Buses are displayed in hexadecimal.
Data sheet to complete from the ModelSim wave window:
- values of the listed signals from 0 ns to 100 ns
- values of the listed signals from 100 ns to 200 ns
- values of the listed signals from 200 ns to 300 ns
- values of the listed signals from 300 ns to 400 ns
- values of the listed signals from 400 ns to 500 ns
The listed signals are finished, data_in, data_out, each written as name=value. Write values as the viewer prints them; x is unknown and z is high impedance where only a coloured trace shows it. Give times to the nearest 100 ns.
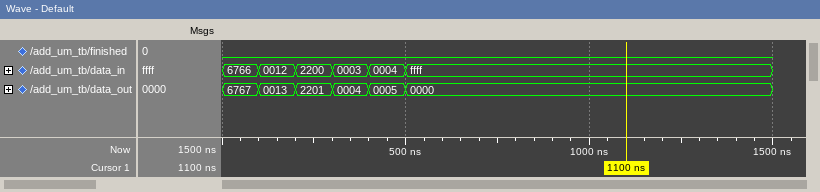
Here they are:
finished=0, data_in=6766, data_out=6767
finished=0, data_in=0012, data_out=0013
finished=0, data_in=2200, data_out=2201
finished=0, data_in=0003, data_out=0004
finished=0, data_in=0004, data_out=0005
